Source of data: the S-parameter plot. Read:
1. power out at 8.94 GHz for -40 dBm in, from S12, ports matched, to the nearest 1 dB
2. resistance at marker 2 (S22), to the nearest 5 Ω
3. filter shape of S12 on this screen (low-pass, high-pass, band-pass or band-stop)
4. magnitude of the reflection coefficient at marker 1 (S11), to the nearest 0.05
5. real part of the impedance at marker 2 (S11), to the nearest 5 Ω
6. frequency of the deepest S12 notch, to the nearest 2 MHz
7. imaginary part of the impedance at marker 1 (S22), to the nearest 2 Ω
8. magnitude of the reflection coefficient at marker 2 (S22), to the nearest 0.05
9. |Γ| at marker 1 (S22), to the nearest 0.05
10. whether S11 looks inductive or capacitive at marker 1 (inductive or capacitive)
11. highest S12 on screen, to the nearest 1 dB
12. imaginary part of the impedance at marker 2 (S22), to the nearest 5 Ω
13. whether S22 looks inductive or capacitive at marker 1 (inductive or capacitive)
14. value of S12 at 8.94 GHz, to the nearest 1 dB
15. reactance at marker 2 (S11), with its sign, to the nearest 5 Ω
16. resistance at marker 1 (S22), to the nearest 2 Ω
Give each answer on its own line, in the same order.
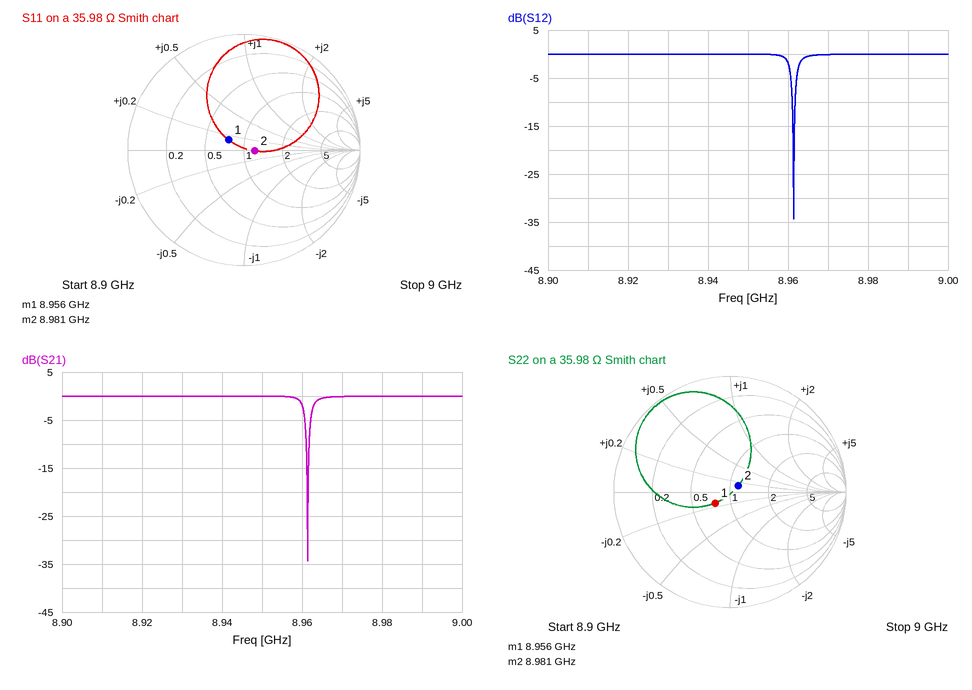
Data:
-40 dBm
40 Ω
band-stop
0.15
45 Ω
8.962 GHz
-6 Ω
0.10
0.15
inductive
0 dB
+5 Ω
capacitive
0 dB
0 Ω
28 Ω
